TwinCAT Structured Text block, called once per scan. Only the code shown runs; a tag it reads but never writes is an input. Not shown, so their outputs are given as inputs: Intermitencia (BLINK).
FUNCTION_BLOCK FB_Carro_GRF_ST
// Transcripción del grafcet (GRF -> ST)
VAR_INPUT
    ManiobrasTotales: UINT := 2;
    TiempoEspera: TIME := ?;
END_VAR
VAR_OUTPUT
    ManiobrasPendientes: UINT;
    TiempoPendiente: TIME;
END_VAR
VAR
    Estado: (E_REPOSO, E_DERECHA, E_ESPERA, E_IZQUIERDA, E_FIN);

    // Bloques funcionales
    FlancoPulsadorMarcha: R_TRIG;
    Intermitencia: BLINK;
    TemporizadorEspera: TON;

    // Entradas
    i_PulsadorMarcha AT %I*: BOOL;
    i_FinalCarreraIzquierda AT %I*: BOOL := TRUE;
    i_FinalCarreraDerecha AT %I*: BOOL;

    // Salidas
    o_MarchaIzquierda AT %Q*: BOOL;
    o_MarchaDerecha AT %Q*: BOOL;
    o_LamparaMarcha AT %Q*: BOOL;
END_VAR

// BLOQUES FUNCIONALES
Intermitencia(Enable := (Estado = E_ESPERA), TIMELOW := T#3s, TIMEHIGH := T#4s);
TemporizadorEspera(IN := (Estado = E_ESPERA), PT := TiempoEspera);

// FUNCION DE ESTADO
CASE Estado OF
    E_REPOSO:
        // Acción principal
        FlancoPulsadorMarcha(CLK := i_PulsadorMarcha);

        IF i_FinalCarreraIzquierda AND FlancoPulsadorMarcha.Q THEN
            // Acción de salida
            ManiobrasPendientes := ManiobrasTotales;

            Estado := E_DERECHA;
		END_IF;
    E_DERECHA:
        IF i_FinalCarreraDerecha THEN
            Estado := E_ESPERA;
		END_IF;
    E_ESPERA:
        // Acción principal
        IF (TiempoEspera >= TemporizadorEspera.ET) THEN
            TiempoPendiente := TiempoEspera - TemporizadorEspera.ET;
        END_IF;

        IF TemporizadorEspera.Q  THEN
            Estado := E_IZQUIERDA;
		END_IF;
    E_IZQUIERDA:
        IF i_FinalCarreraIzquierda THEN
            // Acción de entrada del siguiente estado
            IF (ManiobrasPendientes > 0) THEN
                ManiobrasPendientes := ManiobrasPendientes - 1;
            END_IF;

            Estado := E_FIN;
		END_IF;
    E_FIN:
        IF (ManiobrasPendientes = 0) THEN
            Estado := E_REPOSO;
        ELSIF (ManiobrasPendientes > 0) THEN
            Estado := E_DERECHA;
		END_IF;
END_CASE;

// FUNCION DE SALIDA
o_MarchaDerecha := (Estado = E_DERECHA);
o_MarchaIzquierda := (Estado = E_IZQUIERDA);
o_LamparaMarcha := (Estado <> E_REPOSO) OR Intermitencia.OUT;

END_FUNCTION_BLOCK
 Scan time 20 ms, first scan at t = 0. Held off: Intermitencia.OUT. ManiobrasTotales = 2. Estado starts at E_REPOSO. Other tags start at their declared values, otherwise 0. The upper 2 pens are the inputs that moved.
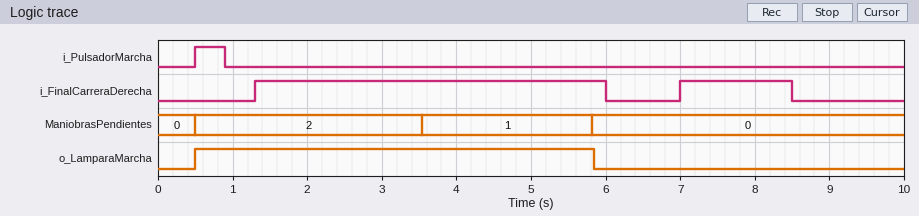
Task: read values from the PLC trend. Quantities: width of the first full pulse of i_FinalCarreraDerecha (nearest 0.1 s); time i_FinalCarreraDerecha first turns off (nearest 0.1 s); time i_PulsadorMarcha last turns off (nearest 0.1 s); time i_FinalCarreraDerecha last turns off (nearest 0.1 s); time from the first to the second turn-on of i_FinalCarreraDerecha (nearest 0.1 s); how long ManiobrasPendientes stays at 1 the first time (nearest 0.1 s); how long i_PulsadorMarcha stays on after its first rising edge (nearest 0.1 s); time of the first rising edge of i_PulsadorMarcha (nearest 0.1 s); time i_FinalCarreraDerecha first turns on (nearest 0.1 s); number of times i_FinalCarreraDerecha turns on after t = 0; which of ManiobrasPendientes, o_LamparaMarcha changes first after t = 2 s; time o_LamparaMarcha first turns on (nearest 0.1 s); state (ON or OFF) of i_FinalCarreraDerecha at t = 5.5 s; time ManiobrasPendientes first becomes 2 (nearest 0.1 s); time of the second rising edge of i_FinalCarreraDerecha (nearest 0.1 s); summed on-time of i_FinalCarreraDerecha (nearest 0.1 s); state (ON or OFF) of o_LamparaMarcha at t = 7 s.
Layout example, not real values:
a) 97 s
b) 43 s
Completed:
a) 4.7 s
b) 6.0 s
c) 0.9 s
d) 8.5 s
e) 5.7 s
f) 2.3 s
g) 0.4 s
h) 0.5 s
i) 1.3 s
j) 2
k) ManiobrasPendientes
l) 0.5 s
m) ON
n) 0.5 s
o) 7.0 s
p) 6.2 s
q) OFF
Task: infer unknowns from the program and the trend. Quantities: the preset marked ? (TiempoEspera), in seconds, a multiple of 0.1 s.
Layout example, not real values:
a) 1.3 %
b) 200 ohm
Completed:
a) 2.2 s
